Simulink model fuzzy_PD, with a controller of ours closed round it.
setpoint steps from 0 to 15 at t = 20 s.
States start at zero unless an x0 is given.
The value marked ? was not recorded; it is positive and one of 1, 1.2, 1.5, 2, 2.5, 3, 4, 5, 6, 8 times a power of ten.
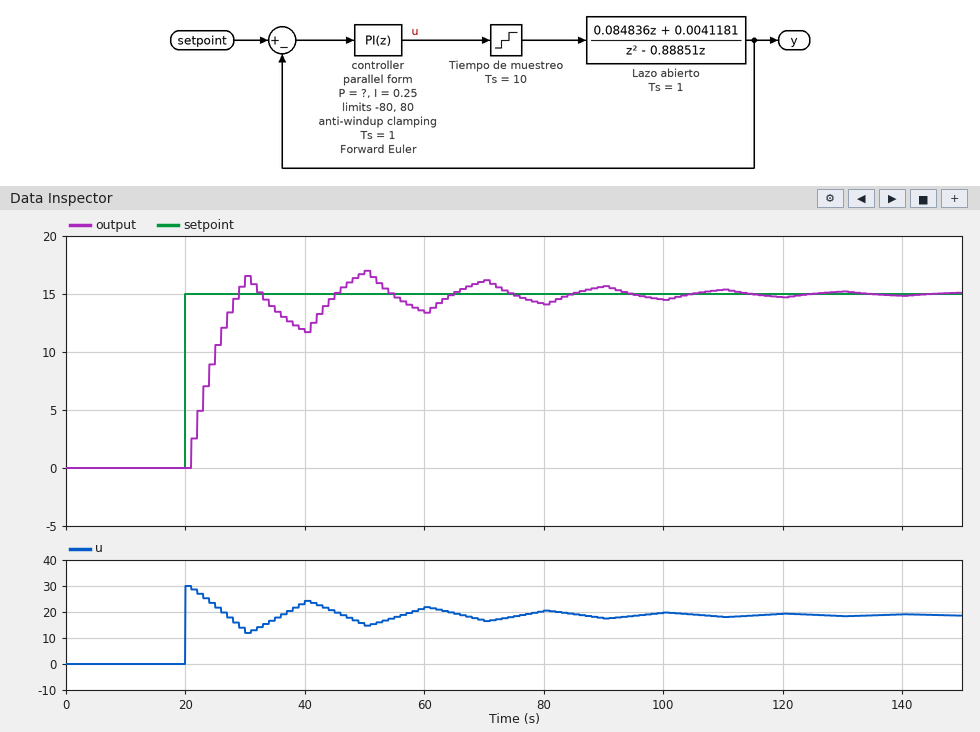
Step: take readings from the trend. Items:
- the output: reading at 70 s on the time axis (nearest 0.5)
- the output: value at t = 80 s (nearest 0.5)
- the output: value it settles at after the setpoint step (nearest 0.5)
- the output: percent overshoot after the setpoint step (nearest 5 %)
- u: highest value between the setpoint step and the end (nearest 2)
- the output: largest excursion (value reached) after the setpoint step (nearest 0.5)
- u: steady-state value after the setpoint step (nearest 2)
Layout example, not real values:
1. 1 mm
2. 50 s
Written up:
1. 16.0
2. 14.0
3. 15.0
4. 15 %
5. 30
6. 17.0
7. 18
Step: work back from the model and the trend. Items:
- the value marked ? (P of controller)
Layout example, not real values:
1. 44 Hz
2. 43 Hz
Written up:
1. 2
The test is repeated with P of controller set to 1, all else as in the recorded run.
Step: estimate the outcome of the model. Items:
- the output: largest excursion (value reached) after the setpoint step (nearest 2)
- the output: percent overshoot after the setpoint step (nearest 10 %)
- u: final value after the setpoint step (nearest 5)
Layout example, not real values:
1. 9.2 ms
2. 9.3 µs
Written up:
1. 20
2. 40 %
3. 20
